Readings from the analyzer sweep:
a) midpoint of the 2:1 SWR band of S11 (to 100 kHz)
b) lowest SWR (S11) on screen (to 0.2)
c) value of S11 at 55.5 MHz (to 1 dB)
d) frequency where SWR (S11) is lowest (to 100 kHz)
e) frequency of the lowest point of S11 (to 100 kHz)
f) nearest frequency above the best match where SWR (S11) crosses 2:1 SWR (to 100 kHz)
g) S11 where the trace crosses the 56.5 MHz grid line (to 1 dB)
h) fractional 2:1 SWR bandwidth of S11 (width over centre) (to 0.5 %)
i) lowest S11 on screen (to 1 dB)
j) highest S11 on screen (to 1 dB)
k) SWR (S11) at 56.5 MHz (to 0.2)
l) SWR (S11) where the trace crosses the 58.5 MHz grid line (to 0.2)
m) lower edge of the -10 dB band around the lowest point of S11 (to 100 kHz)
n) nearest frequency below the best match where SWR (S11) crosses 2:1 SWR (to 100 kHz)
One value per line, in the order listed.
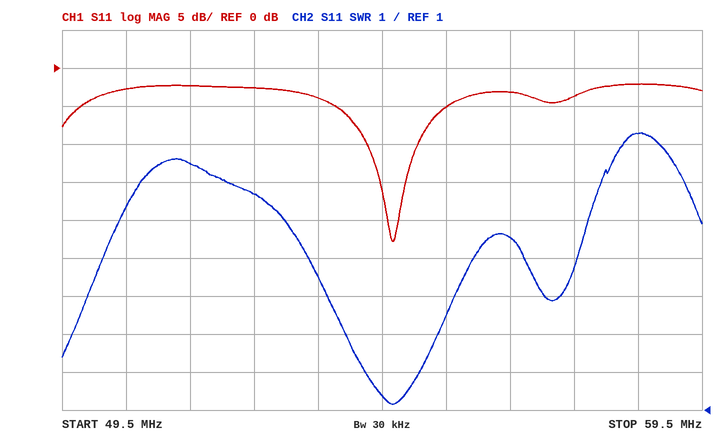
54.7 MHz
1.2
-5 dB
54.7 MHz
54.7 MHz
55.1 MHz
-3 dB
1.5 %
-23 dB
-2 dB
5.6
8.2
54.3 MHz
54.2 MHz
